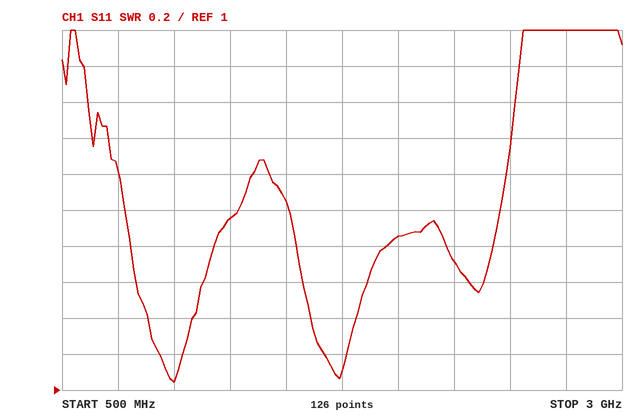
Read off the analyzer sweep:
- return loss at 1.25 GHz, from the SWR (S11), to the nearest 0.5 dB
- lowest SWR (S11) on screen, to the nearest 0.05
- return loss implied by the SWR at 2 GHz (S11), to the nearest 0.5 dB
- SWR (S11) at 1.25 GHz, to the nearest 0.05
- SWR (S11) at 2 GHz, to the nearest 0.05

10.0 dB
1.05
10.5 dB
1.95
1.85
